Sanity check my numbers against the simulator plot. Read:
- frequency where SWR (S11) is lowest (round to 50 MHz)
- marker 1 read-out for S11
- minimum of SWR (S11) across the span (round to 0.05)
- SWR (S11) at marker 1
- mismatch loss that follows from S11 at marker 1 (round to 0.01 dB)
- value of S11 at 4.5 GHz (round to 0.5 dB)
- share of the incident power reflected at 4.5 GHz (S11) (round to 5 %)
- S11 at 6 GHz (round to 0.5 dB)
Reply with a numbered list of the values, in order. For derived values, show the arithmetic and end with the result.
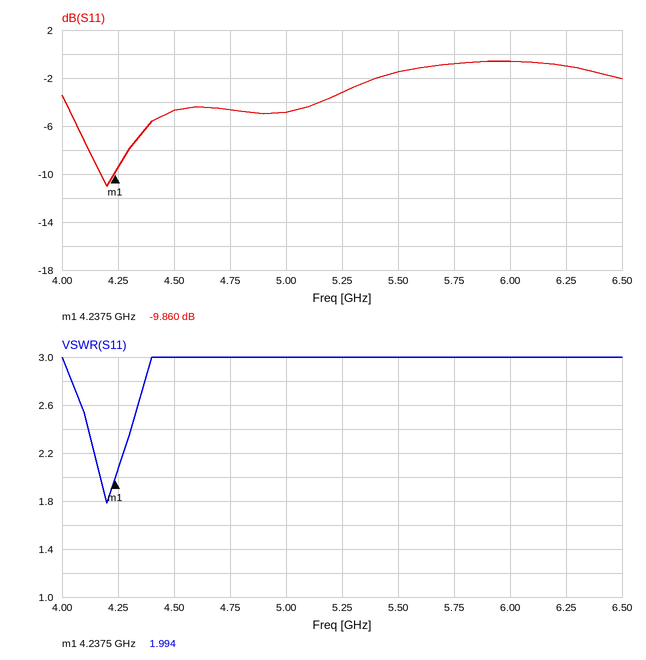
1. 4.20 GHz
2. -9.860 dB
3. 1.80
4. 1.994
5. −10 log10(1 − 10^(-9.86/10)) ≈ 0.47 dB
6. -4.5 dB
7. 10^(-4.5/10) ≈ 35 %
8. -0.5 dB
